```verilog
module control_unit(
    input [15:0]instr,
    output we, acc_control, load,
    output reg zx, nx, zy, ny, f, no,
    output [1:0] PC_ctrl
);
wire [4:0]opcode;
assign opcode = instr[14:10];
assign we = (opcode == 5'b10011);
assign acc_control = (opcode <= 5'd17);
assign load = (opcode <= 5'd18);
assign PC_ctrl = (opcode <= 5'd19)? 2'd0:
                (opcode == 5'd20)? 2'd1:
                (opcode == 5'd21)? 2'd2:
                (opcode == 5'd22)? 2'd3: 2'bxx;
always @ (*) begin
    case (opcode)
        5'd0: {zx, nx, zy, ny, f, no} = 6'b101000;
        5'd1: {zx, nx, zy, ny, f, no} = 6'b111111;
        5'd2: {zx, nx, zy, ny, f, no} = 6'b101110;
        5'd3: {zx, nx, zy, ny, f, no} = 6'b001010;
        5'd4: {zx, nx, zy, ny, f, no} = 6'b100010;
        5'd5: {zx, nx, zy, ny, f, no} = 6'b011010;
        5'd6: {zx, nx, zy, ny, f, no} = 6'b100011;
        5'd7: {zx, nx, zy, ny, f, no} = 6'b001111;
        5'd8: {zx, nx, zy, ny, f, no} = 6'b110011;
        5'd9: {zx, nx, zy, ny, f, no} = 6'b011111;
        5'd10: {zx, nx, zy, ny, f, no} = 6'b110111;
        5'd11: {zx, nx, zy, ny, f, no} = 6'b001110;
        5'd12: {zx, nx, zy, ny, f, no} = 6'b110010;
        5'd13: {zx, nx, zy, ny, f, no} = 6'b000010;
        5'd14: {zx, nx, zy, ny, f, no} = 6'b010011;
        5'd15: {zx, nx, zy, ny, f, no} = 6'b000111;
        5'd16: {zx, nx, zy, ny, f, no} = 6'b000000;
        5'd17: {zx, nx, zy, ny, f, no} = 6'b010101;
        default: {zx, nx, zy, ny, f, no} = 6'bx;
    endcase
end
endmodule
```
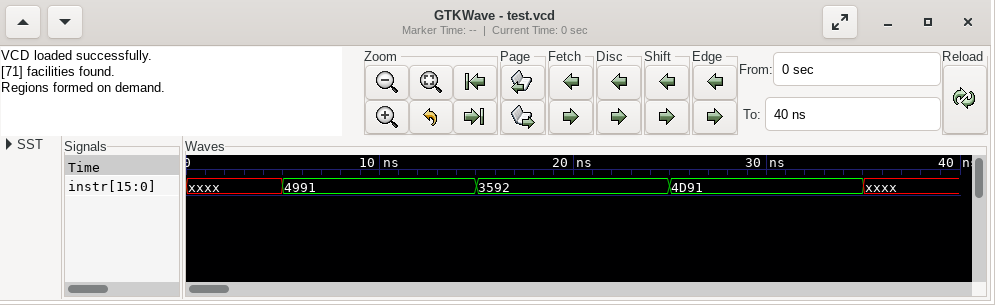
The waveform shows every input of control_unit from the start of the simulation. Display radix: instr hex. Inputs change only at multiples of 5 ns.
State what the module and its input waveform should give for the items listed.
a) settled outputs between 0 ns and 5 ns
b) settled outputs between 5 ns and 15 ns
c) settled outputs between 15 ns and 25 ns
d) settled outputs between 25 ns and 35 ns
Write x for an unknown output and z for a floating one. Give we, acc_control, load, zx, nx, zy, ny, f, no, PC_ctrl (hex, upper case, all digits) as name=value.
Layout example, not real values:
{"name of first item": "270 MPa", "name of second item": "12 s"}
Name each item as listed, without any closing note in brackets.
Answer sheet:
{"settled outputs between 0 ns and 5 ns": "we=x, acc_control=x, load=x, zx=x, nx=x, zy=x, ny=x, f=x, no=x, PC_ctrl=x", "settled outputs between 5 ns and 15 ns": "we=0, acc_control=0, load=1, zx=x, nx=x, zy=x, ny=x, f=x, no=x, PC_ctrl=0", "settled outputs between 15 ns and 25 ns": "we=0, acc_control=1, load=1, zx=0, nx=0, zy=0, ny=0, f=1, no=0, PC_ctrl=0", "settled outputs between 25 ns and 35 ns": "we=1, acc_control=0, load=0, zx=x, nx=x, zy=x, ny=x, f=x, no=x, PC_ctrl=0"}
